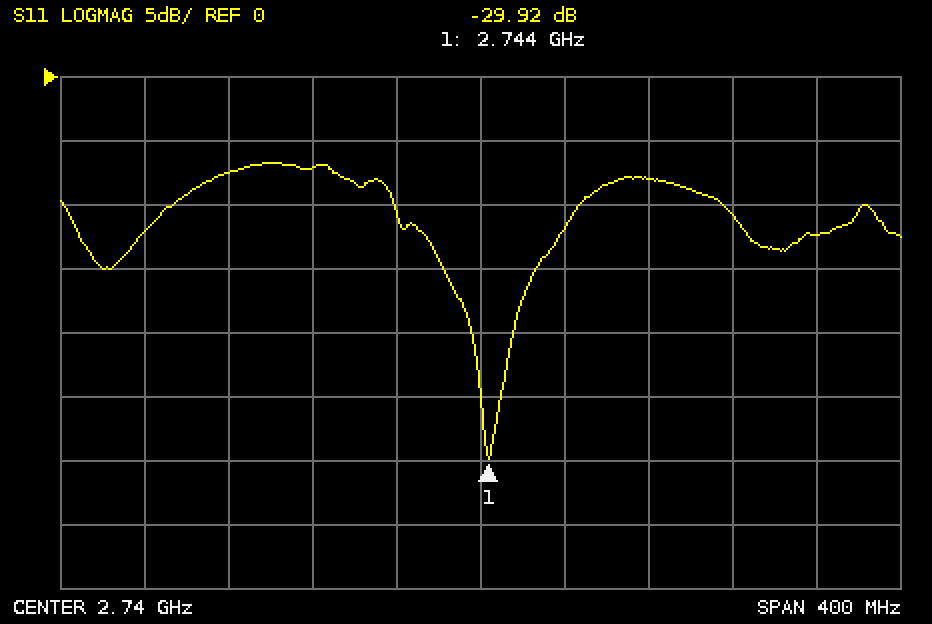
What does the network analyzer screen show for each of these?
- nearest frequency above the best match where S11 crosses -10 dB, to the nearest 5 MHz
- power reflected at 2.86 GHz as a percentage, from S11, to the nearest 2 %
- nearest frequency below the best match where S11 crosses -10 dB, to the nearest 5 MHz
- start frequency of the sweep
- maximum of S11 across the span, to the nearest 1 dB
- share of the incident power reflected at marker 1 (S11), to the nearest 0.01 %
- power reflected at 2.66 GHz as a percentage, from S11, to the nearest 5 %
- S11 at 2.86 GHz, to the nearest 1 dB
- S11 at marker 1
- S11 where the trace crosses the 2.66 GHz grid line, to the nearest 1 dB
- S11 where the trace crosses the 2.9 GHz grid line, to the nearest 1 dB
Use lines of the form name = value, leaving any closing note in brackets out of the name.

nearest frequency above the best match where S11 crosses -10 dB, to the nearest 5 MHz = 2.785 GHz
power reflected at 2.86 GHz as a percentage, from S11, to the nearest 2 % = 8 %
nearest frequency below the best match where S11 crosses -10 dB, to the nearest 5 MHz = 2.700 GHz
start frequency of the sweep = 2.54 GHz
maximum of S11 across the span, to the nearest 1 dB = -7 dB
share of the incident power reflected at marker 1 (S11), to the nearest 0.01 % = 0.10 %
power reflected at 2.66 GHz as a percentage, from S11, to the nearest 5 % = 20 %
S11 at 2.86 GHz, to the nearest 1 dB = -11 dB
S11 at marker 1 = -29.92 dB
S11 where the trace crosses the 2.66 GHz grid line, to the nearest 1 dB = -7 dB
S11 where the trace crosses the 2.9 GHz grid line, to the nearest 1 dB = -12 dB
